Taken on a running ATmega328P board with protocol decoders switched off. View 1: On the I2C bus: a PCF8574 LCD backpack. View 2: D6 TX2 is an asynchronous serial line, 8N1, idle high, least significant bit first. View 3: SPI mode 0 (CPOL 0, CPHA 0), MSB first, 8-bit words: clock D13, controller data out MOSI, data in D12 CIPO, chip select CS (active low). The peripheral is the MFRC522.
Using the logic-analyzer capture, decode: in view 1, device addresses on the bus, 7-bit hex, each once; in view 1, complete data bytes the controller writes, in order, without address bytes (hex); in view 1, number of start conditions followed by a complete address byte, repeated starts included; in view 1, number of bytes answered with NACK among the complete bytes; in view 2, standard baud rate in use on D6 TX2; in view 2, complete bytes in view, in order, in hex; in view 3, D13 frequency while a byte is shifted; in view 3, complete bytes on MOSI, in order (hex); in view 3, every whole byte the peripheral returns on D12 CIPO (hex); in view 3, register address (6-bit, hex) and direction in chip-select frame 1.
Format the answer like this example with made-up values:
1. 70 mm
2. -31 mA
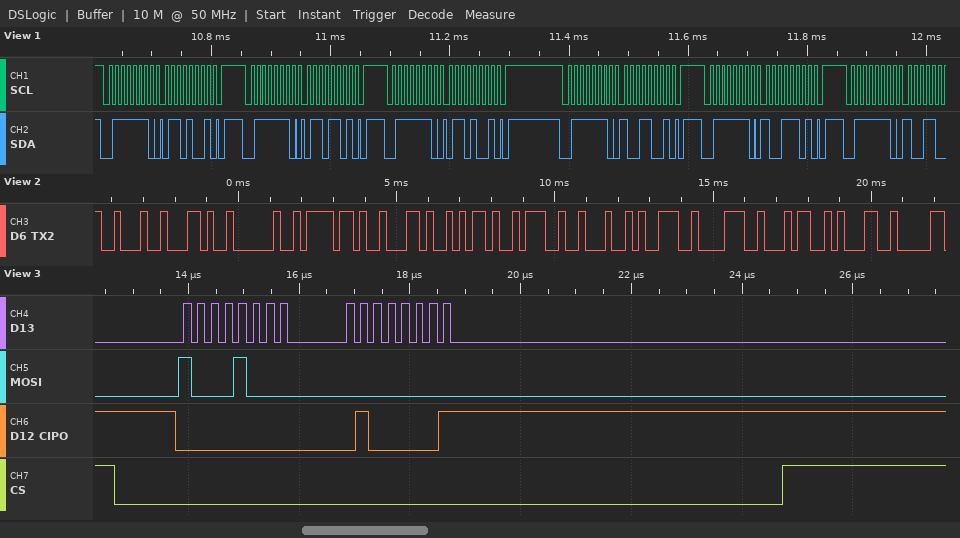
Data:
1. 0x3F
2. 69 6D 69 99 9D
3. 6
4. 0
5. 4800 baud
6. 0x22 0x2C 0x20 0x6F 0x62 0x6A 0x3A 0x22 0x39 0x38 0x34 0x31
7. 4 MHz
8. 88 00
9. 00 41
10. 0x04 read
